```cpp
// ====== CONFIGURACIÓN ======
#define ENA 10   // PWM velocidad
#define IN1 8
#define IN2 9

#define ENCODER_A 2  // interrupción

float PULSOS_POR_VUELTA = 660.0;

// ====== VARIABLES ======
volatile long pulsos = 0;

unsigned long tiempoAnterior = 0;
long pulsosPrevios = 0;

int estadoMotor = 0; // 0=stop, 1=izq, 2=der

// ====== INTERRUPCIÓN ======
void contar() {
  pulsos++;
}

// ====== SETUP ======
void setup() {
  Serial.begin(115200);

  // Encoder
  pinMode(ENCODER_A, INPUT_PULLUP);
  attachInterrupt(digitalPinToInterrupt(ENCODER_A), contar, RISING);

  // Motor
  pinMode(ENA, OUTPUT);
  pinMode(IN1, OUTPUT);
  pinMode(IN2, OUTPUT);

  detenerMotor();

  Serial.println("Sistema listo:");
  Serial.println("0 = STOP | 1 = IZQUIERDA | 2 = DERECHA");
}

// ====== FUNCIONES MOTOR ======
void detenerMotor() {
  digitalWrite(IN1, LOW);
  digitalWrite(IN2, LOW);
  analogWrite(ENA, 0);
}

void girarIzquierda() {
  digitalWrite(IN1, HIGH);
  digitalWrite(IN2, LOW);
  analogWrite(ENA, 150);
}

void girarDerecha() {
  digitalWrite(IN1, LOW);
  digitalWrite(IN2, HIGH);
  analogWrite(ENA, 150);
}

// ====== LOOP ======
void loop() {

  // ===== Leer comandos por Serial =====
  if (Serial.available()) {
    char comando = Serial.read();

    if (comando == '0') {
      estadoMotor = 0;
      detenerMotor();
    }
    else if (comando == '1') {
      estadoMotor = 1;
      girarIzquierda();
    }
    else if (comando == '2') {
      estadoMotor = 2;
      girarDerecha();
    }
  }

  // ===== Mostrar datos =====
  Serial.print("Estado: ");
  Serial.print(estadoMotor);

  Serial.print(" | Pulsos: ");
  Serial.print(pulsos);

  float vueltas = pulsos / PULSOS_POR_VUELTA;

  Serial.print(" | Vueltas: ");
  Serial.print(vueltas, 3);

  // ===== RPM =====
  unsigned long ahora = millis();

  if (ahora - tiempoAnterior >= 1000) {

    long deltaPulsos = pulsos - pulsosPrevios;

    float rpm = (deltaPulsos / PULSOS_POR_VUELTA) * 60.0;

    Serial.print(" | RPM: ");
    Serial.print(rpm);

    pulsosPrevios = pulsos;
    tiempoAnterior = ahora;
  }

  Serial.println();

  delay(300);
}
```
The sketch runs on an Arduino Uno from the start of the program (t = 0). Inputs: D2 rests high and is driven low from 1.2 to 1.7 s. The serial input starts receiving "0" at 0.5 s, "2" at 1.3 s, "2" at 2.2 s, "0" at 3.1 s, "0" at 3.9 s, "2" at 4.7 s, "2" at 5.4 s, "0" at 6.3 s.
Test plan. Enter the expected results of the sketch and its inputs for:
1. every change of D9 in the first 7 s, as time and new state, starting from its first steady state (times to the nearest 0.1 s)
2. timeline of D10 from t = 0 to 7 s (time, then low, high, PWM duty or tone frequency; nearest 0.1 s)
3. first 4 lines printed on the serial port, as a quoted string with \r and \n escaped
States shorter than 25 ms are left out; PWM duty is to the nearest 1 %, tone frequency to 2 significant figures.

0 s low; 1.5 s high; 3.3 s low; 4.8 s high; 6.3 s low
0 s low; 1.5 s PWM 59 %; 3.3 s low; 4.8 s PWM 59 %; 6.3 s low
"Sistema listo:\r\n0 = STOP | 1 = IZQUIERDA | 2 = DERECHA\r\nEstado: 0 | Pulsos: 0 | Vueltas: 0.000\r\nEstado: 0 | Pulsos: 0 | Vueltas: 0.000\r\n"
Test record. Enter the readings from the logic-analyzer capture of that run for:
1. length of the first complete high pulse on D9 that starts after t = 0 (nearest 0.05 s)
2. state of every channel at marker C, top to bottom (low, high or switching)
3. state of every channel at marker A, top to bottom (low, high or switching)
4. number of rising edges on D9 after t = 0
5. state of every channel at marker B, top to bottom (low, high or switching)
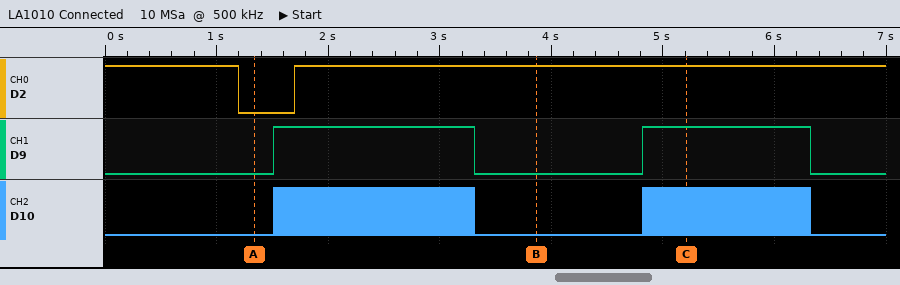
1.80 s
D2 high, D9 high, D10 switching
D2 low, D9 low, D10 low
2
D2 high, D9 low, D10 low
